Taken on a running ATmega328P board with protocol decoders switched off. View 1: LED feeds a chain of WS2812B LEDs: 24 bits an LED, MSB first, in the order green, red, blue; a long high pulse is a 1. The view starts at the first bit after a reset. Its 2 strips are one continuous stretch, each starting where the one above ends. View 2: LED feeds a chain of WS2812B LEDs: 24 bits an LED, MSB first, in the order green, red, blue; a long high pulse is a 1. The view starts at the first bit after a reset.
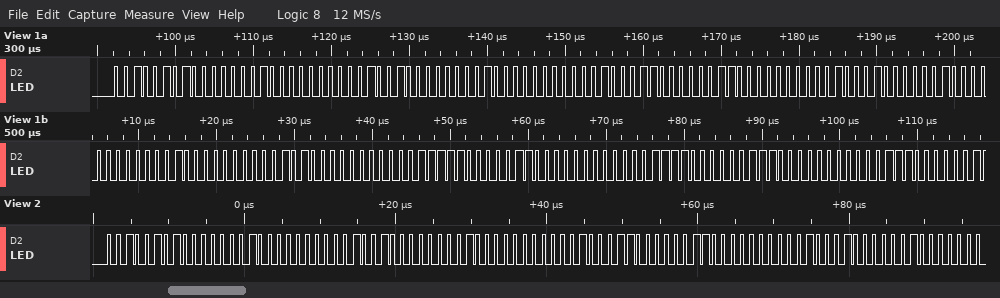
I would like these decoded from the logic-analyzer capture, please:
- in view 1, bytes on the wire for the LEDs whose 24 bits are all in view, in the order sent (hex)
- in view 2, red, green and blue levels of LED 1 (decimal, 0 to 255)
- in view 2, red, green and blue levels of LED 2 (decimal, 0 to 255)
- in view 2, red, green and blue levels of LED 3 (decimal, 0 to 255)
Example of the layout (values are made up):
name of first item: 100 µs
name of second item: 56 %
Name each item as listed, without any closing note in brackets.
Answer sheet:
in view 1, bytes on the wire for the LEDs whose 24 bits are all in view, in the order sent: 25 01 00 24 02 00 23 03 00 22 04 00 20 05 00 1F 06 00 1E 07 00
in view 2, red, green and blue levels of LED 1: 1, 37, 0
in view 2, red, green and blue levels of LED 2: 2, 36, 0
in view 2, red, green and blue levels of LED 3: 3, 35, 0
